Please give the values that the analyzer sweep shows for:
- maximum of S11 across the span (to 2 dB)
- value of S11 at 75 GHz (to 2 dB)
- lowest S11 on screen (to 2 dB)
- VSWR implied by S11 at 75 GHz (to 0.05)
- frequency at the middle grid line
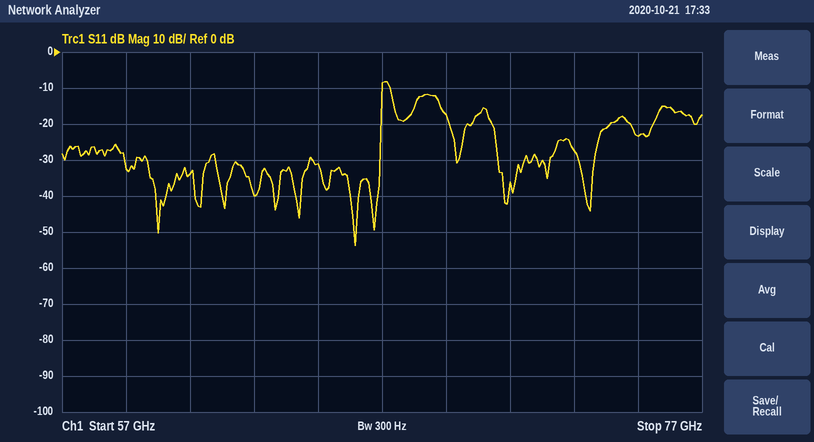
-8 dB
-24 dB
-54 dB
1.15
67 GHz
